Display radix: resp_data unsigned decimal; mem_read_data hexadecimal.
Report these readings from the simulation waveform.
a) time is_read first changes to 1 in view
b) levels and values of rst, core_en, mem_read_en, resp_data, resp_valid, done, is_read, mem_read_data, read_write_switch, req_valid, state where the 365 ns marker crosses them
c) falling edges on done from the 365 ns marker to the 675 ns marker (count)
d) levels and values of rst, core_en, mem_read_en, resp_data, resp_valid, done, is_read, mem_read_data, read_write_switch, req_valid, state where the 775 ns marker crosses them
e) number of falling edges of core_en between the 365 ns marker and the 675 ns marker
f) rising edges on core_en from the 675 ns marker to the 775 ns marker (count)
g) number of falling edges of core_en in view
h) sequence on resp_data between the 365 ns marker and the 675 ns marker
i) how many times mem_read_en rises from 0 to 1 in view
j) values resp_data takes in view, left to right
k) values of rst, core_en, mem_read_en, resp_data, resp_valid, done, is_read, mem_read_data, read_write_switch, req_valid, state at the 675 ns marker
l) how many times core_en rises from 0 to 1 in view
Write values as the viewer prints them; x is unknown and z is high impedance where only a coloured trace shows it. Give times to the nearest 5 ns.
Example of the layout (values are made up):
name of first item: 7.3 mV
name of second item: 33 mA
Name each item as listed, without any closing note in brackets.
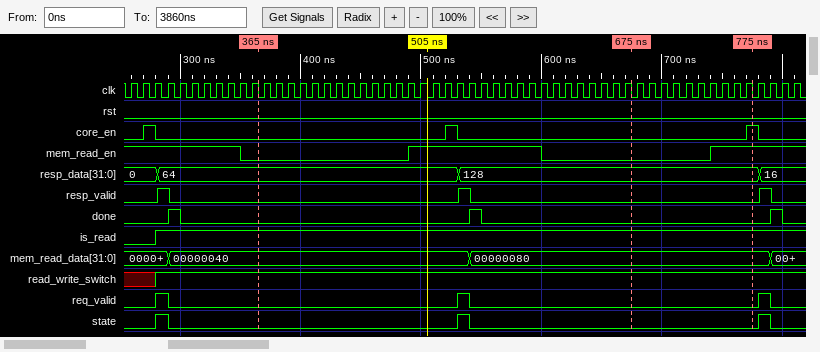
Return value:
time is_read first changes to 1 in view: 280 ns
levels and values of rst, core_en, mem_read_en, resp_data, resp_valid, done, is_read, mem_read_data, read_write_switch, req_valid, state where the 365 ns marker crosses them: rst=0, core_en=0, mem_read_en=0, resp_data=64, resp_valid=0, done=0, is_read=1, mem_read_data=00000040, read_write_switch=1, req_valid=0, state=0
falling edges on done from the 365 ns marker to the 675 ns marker: 1
levels and values of rst, core_en, mem_read_en, resp_data, resp_valid, done, is_read, mem_read_data, read_write_switch, req_valid, state where the 775 ns marker crosses them: rst=0, core_en=1, mem_read_en=1, resp_data=128, resp_valid=0, done=0, is_read=1, mem_read_data=00000080, read_write_switch=1, req_valid=0, state=0
number of falling edges of core_en between the 365 ns marker and the 675 ns marker: 1
rising edges on core_en from the 675 ns marker to the 775 ns marker: 1
number of falling edges of core_en in view: 3
sequence on resp_data between the 365 ns marker and the 675 ns marker: 64, 128
how many times mem_read_en rises from 0 to 1 in view: 2
values resp_data takes in view, left to right: 0, 64, 128, 16
values of rst, core_en, mem_read_en, resp_data, resp_valid, done, is_read, mem_read_data, read_write_switch, req_valid, state at the 675 ns marker: rst=0, core_en=0, mem_read_en=0, resp_data=128, resp_valid=0, done=0, is_read=1, mem_read_data=00000080, read_write_switch=1, req_valid=0, state=0
how many times core_en rises from 0 to 1 in view: 3
